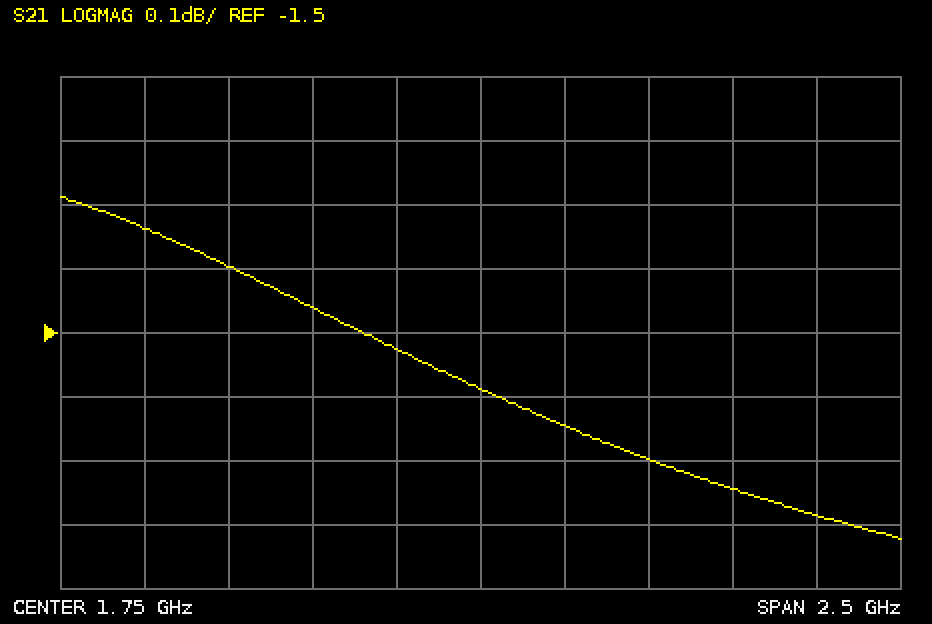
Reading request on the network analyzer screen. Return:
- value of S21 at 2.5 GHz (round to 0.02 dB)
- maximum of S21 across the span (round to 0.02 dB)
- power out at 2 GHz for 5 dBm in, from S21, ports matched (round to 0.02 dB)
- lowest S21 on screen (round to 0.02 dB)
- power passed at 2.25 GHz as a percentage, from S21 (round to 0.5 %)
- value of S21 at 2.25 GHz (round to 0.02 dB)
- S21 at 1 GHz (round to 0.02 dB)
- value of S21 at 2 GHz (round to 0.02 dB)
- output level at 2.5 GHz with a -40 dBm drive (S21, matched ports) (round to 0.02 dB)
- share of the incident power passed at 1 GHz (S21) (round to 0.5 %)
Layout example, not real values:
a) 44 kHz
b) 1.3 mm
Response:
a) -1.74 dB
b) -1.28 dB
c) 3.36 dBm
d) -1.82 dB
e) 67.5 %
f) -1.70 dB
g) -1.40 dB
h) -1.64 dB
i) -41.74 dBm
j) 72.5 %
